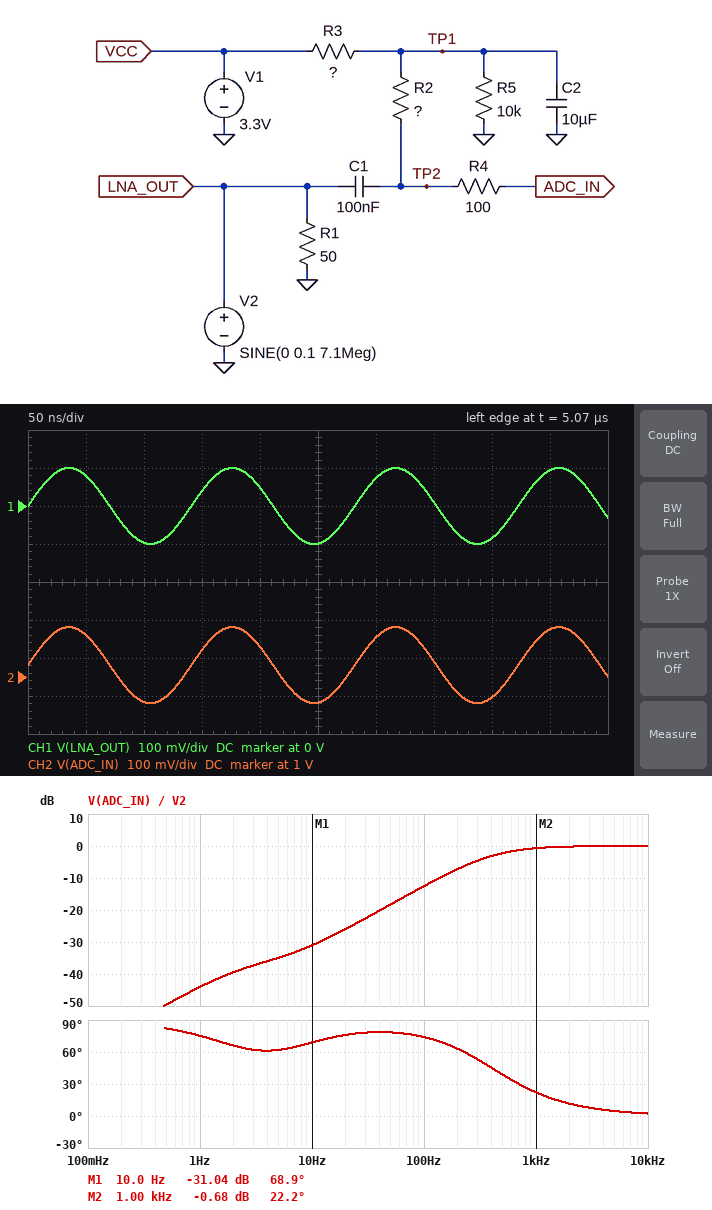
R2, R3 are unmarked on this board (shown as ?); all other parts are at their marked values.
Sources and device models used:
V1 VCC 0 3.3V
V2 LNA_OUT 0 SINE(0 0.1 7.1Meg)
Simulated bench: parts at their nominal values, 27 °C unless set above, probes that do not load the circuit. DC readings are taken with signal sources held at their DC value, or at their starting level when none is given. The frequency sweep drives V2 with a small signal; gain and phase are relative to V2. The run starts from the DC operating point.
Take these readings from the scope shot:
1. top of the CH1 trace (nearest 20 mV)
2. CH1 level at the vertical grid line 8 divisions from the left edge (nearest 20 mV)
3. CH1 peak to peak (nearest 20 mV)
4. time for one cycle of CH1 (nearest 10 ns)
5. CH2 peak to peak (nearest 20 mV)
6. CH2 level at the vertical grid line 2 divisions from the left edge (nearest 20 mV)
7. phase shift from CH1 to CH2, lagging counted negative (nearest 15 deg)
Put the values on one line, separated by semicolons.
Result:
100 mV; -80 mV; 200 mV; 140 ns; 200 mV; 940 mV; 0 deg
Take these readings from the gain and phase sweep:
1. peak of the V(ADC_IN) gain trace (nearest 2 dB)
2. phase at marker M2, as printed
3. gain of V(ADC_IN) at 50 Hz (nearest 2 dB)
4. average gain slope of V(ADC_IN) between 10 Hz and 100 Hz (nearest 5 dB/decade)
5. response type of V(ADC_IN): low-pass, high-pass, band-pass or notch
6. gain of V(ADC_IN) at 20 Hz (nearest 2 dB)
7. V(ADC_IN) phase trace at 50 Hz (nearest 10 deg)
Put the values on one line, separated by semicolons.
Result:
0 dB; 22.2 deg; -18 dB; 20 dB/decade; high-pass; -26 dB; 80 deg
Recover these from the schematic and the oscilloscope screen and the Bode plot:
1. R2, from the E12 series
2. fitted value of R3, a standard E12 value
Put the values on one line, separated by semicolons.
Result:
3.9 kΩ; 22 kΩ
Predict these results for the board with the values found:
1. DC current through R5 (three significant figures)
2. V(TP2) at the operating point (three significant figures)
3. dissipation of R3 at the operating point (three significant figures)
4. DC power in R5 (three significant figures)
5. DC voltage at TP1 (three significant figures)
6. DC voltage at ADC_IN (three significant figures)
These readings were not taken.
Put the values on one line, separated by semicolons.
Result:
103 µA; 1.03 V; 234 µW; 106 µW; 1.03 V; 1.03 V
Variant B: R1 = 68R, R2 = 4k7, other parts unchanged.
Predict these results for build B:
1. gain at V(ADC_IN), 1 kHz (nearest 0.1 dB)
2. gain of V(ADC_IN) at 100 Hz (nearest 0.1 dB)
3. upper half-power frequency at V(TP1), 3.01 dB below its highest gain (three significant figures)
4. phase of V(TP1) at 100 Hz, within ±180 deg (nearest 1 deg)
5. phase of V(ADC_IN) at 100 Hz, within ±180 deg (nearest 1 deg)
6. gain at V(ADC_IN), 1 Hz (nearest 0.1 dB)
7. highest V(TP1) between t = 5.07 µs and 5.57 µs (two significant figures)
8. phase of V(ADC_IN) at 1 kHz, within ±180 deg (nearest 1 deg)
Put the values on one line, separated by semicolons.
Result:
-0.5 dB; -11.0 dB; 347 Hz; -15 deg; 72 deg; -43.4 dB; 1.0 V; 19 deg
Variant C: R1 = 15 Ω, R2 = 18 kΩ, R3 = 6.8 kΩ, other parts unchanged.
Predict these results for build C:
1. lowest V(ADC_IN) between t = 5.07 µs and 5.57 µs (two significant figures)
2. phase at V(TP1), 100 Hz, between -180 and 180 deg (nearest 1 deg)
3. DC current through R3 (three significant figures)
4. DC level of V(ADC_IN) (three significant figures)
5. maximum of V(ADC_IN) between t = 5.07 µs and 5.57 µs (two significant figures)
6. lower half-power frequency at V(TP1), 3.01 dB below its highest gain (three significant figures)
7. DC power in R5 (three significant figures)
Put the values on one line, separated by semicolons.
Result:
1.9 V; -46 deg; 196 µA; 1.96 V; 2.1 V; 3.59 Hz; 386 µW
